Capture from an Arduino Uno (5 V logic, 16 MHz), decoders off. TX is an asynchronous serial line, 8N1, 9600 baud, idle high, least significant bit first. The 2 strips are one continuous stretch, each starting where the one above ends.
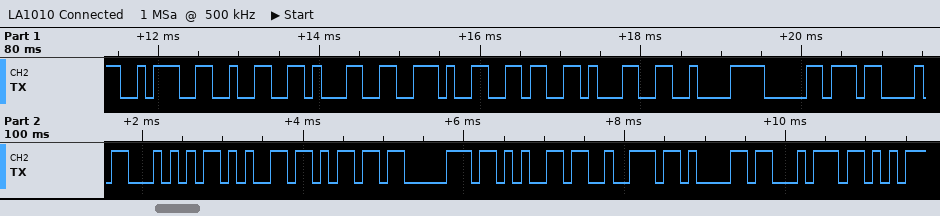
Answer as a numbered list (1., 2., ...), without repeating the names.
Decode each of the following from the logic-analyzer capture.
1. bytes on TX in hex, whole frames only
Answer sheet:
1. 0x3A 0x32 0x31 0x2E 0x36 0x31 0xC2 0xB0 0x43 0x54 0x65 0x6D 0x70 0x65 0x72 0x61 0x74
